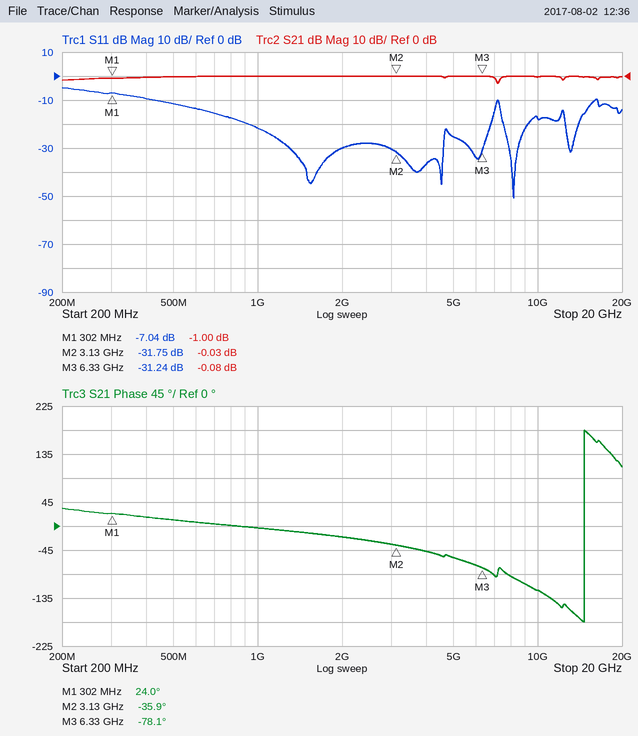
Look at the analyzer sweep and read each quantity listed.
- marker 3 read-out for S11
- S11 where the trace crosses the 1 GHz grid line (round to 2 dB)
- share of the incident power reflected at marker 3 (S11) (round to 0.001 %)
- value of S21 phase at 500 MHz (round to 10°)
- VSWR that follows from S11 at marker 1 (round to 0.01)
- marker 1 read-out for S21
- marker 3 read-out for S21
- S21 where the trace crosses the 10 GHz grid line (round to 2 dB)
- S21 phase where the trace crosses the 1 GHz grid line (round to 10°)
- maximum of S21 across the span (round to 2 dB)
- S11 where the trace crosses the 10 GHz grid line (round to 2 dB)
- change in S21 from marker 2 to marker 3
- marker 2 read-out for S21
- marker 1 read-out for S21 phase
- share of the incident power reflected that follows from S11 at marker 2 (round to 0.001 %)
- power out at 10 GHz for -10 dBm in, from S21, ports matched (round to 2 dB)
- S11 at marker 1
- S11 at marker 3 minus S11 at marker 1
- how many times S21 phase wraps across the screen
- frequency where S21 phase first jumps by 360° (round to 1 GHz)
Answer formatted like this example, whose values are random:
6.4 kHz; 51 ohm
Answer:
-31.24 dB; -22 dB; 0.075 %; 10°; 2.60; -1.00 dB; -0.08 dB; 0 dB; 0°; 0 dB; -18 dB; -0.05 dB; -0.03 dB; 24.0°; 0.067 %; -10 dBm; -7.04 dB; -24.20 dB; 1; 15 GHz
